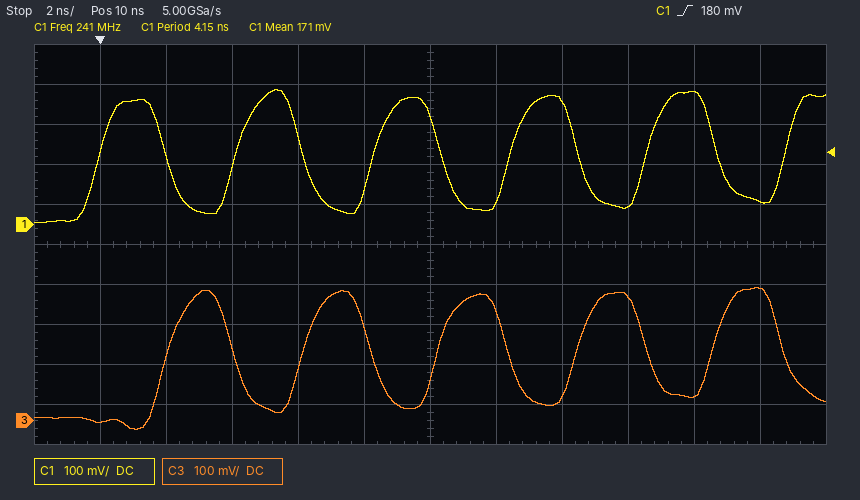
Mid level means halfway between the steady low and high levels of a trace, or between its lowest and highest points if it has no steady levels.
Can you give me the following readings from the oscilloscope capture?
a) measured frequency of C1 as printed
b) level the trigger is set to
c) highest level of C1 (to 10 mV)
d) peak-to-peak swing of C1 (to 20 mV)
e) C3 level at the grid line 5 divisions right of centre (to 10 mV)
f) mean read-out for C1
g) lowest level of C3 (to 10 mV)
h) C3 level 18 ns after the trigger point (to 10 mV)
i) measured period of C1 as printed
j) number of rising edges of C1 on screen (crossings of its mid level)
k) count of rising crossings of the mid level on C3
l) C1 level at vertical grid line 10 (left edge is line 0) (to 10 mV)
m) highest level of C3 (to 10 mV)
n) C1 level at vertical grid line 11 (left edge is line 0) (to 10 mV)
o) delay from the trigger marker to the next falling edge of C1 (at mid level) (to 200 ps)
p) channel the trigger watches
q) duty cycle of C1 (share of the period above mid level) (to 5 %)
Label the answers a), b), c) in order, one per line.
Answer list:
a) 241 MHz
b) 180 mV
c) 340 mV
d) 340 mV
e) 330 mV
f) 171 mV
g) -20 mV
h) 60 mV
i) 4.15 ns
j) 6
k) 5
l) 330 mV
m) 330 mV
n) 60 mV
o) 2.0 ns
p) C1
q) 50 %
